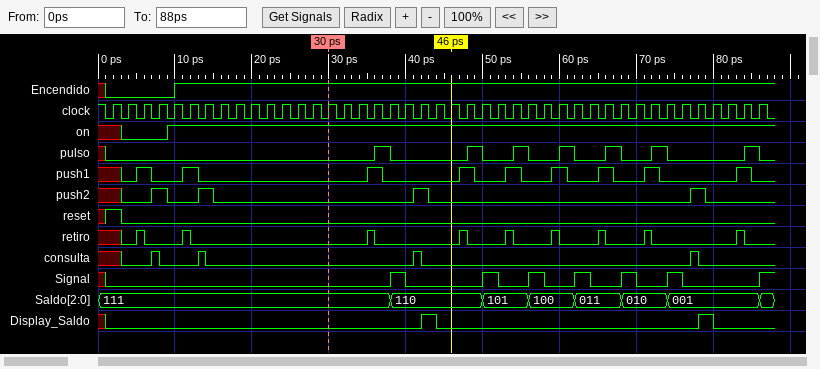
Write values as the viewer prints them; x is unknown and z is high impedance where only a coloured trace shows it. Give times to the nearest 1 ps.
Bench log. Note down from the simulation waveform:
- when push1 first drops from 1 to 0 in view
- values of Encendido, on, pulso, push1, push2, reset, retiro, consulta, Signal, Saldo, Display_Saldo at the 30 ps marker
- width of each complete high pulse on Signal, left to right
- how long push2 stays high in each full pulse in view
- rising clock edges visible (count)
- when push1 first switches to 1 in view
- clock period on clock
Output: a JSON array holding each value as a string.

["7 ps", "Encendido=1, on=1, pulso=0, push1=0, push2=0, reset=0, retiro=0, consulta=0, Signal=0, Saldo=111, Display_Saldo=0", "2 ps, 2 ps, 2 ps, 2 ps, 2 ps, 2 ps", "2 ps, 2 ps, 2 ps, 2 ps", "43", "5 ps", "2 ps"]
